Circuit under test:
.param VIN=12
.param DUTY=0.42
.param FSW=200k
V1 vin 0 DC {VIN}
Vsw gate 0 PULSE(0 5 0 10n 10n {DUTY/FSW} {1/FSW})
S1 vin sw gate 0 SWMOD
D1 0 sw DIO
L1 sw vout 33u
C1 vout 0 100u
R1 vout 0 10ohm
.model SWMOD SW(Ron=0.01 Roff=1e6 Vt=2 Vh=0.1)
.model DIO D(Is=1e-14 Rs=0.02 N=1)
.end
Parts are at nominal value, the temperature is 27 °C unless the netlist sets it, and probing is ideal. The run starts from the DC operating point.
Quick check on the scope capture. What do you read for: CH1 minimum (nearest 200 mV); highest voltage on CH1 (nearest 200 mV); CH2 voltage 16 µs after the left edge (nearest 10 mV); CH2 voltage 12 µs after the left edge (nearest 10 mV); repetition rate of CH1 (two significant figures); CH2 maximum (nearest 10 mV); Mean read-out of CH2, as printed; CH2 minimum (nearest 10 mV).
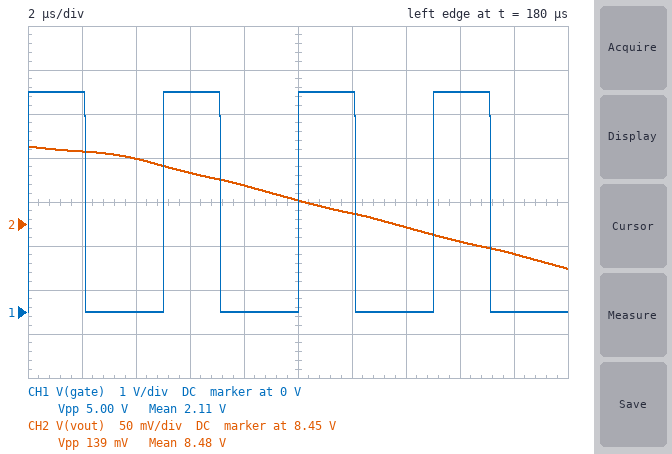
0 V
5.0 V
8.43 V
8.46 V
200 kHz
8.54 V
8.48 V
8.40 V
